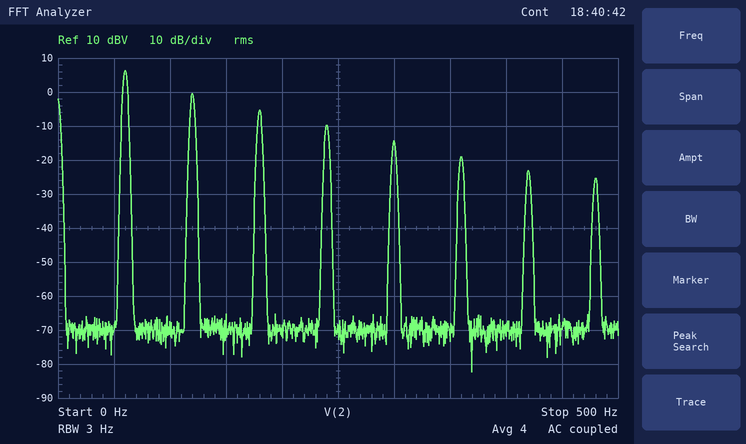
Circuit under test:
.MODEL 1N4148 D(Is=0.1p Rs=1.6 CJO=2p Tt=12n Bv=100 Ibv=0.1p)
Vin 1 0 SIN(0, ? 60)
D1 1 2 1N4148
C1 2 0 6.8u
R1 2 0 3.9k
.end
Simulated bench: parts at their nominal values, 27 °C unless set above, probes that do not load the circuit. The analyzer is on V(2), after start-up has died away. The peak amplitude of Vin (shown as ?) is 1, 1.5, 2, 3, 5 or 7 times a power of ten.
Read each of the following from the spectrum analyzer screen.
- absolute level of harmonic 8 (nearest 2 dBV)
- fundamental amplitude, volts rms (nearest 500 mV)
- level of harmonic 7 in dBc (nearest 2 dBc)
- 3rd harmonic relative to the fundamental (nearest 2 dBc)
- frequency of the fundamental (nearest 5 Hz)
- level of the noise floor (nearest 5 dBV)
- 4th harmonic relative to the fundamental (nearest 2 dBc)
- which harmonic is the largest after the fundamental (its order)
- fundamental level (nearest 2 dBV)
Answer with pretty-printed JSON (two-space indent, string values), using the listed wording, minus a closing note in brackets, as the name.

{
  "absolute level of harmonic 8": "-26 dBV",
  "fundamental amplitude, volts rms": "2.0 V",
  "level of harmonic 7 in dBc": "-30 dBc",
  "3rd harmonic relative to the fundamental": "-12 dBc",
  "frequency of the fundamental": "60 Hz",
  "level of the noise floor": "-70 dBV",
  "4th harmonic relative to the fundamental": "-16 dBc",
  "which harmonic is the largest after the fundamental": "2",
  "fundamental level": "6 dBV"
}
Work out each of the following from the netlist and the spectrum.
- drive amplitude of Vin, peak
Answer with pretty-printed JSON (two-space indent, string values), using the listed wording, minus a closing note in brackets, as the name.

{
  "drive amplitude of Vin, peak": "20 V"
}
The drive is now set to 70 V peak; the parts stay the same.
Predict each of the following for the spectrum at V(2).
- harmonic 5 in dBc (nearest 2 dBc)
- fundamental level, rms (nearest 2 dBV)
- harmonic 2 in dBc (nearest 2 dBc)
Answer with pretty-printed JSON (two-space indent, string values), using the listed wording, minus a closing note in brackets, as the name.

{
  "harmonic 5 in dBc": "-24 dBc",
  "fundamental level, rms": "24 dBV",
  "harmonic 2 in dBc": "-16 dBc"
}
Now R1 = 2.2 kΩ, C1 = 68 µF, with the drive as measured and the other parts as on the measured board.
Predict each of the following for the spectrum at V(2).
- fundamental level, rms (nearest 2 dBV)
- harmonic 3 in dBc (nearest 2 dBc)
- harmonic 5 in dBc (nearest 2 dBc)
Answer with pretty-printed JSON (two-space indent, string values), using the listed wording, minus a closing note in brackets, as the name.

{
  "fundamental level, rms": "-6 dBV",
  "harmonic 3 in dBc": "-10 dBc",
  "harmonic 5 in dBc": "-16 dBc"
}
